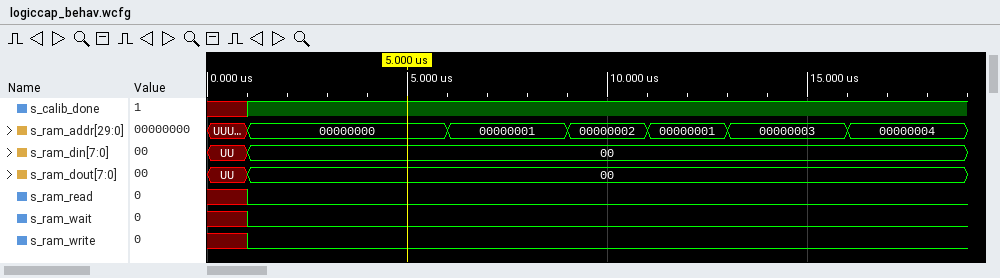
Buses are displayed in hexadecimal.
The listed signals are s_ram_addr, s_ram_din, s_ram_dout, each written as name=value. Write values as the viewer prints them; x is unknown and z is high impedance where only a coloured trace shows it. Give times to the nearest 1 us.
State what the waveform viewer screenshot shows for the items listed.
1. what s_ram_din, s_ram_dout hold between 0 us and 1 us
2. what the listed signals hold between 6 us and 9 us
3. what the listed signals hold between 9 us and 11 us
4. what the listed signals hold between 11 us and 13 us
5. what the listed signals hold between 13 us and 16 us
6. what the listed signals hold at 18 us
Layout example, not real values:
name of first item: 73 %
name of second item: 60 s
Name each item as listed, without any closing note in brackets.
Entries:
what s_ram_din, s_ram_dout hold between 0 us and 1 us: s_ram_din=UU, s_ram_dout=UU
what the listed signals hold between 6 us and 9 us: s_ram_addr=00000001, s_ram_din=00, s_ram_dout=00
what the listed signals hold between 9 us and 11 us: s_ram_addr=00000002, s_ram_din=00, s_ram_dout=00
what the listed signals hold between 11 us and 13 us: s_ram_addr=00000001, s_ram_din=00, s_ram_dout=00
what the listed signals hold between 13 us and 16 us: s_ram_addr=00000003, s_ram_din=00, s_ram_dout=00
what the listed signals hold at 18 us: s_ram_addr=00000004, s_ram_din=00, s_ram_dout=00
